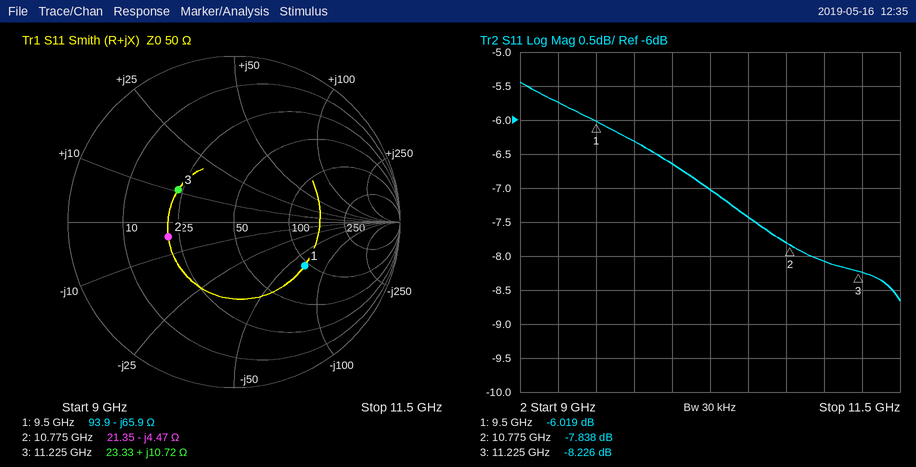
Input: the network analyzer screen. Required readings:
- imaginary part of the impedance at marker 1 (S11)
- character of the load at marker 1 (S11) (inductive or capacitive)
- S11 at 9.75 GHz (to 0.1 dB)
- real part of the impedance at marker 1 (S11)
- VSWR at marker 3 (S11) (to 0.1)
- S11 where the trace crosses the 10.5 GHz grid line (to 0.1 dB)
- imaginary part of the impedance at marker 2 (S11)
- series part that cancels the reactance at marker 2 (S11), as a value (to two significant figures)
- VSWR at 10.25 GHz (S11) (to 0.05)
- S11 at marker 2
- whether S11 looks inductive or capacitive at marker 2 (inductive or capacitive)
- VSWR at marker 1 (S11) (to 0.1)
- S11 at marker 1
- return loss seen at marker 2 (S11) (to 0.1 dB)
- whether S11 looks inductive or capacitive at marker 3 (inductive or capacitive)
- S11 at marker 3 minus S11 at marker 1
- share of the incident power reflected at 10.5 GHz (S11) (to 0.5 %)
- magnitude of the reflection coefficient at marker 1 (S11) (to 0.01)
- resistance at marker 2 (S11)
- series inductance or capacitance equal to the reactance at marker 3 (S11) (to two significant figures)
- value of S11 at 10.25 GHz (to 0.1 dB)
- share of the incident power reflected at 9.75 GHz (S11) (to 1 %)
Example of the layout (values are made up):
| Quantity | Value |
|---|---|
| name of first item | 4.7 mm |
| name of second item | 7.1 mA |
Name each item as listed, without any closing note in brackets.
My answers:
| Quantity | Value |
|---|---|
| imaginary part of the impedance at marker 1 | -65.9 Ω |
| character of the load at marker 1 (S11) | capacitive |
| S11 at 9.75 GHz | -6.3 dB |
| real part of the impedance at marker 1 | 93.9 Ω |
| VSWR at marker 3 (S11) | 2.3 |
| S11 where the trace crosses the 10.5 GHz grid line | -7.4 dB |
| imaginary part of the impedance at marker 2 | -4.47 Ω |
| series part that cancels the reactance at marker 2 (S11), as a value | 66 pH |
| VSWR at 10.25 GHz (S11) | 2.60 |
| S11 at marker 2 | -7.838 dB |
| whether S11 looks inductive or capacitive at marker 2 | capacitive |
| VSWR at marker 1 (S11) | 3.0 |
| S11 at marker 1 | -6.019 dB |
| return loss seen at marker 2 (S11) | 7.8 dB |
| whether S11 looks inductive or capacitive at marker 3 | inductive |
| S11 at marker 3 minus S11 at marker 1 | -2.207 dB |
| share of the incident power reflected at 10.5 GHz (S11) | 18.0 % |
| magnitude of the reflection coefficient at marker 1 (S11) | 0.50 |
| resistance at marker 2 | 21.35 Ω |
| series inductance or capacitance equal to the reactance at marker 3 (S11) | 150 pH |
| value of S11 at 10.25 GHz | -7.0 dB |
| share of the incident power reflected at 9.75 GHz (S11) | 23 % |
